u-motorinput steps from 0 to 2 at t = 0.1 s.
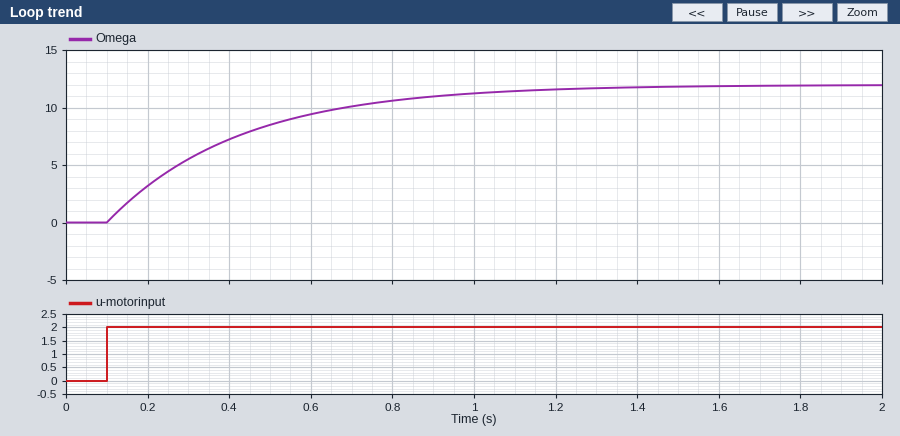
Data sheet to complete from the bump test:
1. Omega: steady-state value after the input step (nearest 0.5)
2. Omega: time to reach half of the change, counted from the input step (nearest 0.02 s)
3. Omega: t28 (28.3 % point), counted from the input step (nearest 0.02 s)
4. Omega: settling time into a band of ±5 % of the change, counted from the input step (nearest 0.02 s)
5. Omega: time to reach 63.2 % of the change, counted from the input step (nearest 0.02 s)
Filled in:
12.0
0.22 s
0.10 s
0.98 s
0.32 s
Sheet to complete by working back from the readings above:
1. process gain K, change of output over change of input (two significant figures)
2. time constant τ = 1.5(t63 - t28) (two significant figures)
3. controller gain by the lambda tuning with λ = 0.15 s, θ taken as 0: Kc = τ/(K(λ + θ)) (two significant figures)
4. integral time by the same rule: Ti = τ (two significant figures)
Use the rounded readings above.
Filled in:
6.0
0.33 s
0.37
0.33 s
